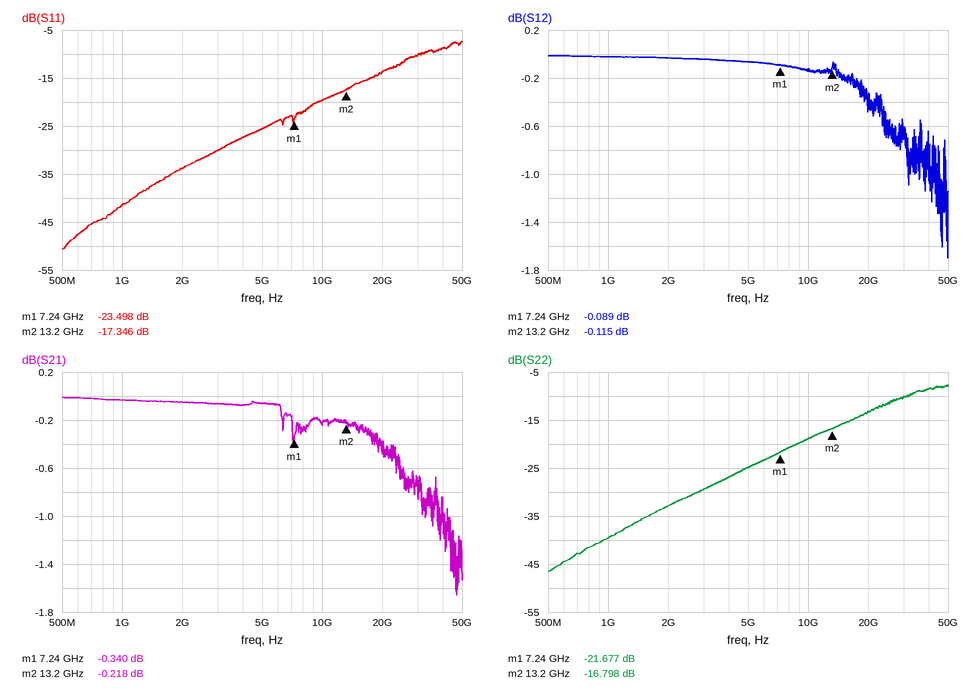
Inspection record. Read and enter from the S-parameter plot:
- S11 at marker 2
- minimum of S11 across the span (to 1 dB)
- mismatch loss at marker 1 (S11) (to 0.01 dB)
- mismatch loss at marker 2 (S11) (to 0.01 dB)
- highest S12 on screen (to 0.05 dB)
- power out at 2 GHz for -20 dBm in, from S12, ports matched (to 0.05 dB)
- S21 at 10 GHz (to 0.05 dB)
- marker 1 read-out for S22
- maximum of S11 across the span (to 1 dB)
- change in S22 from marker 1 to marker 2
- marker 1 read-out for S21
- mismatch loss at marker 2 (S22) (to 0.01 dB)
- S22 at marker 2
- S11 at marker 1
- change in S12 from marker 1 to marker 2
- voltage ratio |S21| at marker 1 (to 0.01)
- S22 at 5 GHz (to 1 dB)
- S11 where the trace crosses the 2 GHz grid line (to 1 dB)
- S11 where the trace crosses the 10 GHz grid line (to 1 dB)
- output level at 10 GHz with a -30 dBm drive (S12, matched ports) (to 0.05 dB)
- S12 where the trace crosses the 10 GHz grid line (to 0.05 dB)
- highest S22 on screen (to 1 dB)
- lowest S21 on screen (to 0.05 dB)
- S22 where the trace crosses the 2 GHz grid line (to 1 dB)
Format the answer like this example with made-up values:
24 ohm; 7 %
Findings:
-17.346 dB; -51 dB; 0.02 dB; 0.08 dB; 0.00 dB; -20.05 dBm; -0.25 dB; -21.677 dB; -7 dB; 4.879 dB; -0.340 dB; 0.09 dB; -16.798 dB; -23.498 dB; -0.026 dB; 0.96; -25 dB; -34 dB; -20 dB; -30.15 dBm; -0.15 dB; -8 dB; -1.65 dB; -33 dB
